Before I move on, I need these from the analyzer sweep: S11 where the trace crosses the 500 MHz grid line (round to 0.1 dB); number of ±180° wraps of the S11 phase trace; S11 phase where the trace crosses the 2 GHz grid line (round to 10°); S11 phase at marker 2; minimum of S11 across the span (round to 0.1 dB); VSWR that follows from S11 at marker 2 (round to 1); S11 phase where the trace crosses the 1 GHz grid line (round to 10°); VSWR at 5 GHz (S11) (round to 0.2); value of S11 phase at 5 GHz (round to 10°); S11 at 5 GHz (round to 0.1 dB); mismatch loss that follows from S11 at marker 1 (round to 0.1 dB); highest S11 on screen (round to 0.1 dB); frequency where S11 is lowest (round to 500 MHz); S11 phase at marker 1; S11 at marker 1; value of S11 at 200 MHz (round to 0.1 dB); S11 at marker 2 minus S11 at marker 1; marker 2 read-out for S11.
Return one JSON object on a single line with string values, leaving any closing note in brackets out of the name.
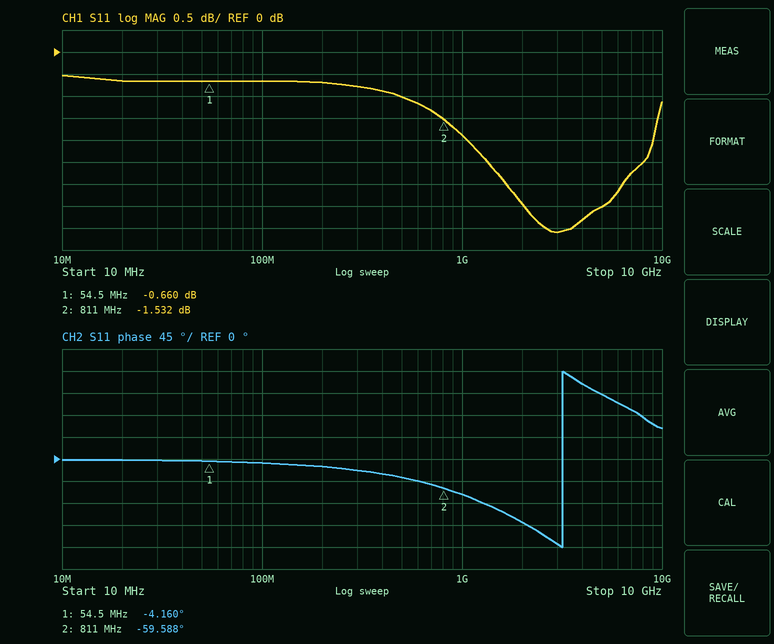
{"S11 where the trace crosses the 500 MHz grid line": "-1.0 dB", "number of ±180° wraps of the S11 phase trace": "1", "S11 phase where the trace crosses the 2 GHz grid line": "-130°", "S11 phase at marker 2": "-59.588°", "minimum of S11 across the span": "-4.1 dB", "VSWR that follows from S11 at marker 2": "11", "S11 phase where the trace crosses the 1 GHz grid line": "-70°", "VSWR at 5 GHz (S11)": "5.0", "value of S11 phase at 5 GHz": "130°", "S11 at 5 GHz": "-3.5 dB", "mismatch loss that follows from S11 at marker 1": "8.5 dB", "highest S11 on screen": "-0.5 dB", "frequency where S11 is lowest": "3.0 GHz", "S11 phase at marker 1": "-4.160°", "S11 at marker 1": "-0.660 dB", "value of S11 at 200 MHz": "-0.7 dB", "S11 at marker 2 minus S11 at marker 1": "-0.872 dB", "marker 2 read-out for S11": "-1.532 dB"}
